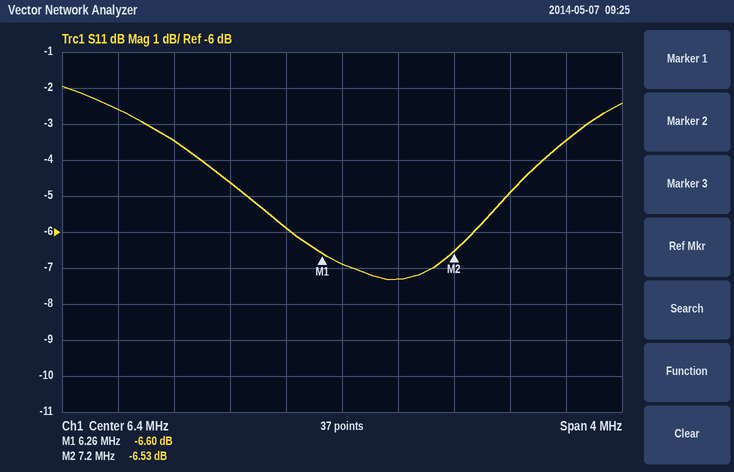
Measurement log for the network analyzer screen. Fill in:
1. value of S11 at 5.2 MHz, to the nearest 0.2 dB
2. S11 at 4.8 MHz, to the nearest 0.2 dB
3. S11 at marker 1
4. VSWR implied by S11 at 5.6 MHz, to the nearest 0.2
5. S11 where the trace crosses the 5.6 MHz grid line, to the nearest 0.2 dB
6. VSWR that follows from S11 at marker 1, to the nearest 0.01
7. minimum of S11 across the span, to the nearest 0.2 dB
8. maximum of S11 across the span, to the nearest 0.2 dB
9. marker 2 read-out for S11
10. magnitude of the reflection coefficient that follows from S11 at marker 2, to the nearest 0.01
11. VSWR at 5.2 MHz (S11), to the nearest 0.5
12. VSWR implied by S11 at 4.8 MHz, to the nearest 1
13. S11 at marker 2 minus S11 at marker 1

-3.4 dB
-2.6 dB
-6.60 dB
3.8
-4.6 dB
2.76
-7.4 dB
-2.0 dB
-6.53 dB
0.47
5.0
7
0.07 dB
